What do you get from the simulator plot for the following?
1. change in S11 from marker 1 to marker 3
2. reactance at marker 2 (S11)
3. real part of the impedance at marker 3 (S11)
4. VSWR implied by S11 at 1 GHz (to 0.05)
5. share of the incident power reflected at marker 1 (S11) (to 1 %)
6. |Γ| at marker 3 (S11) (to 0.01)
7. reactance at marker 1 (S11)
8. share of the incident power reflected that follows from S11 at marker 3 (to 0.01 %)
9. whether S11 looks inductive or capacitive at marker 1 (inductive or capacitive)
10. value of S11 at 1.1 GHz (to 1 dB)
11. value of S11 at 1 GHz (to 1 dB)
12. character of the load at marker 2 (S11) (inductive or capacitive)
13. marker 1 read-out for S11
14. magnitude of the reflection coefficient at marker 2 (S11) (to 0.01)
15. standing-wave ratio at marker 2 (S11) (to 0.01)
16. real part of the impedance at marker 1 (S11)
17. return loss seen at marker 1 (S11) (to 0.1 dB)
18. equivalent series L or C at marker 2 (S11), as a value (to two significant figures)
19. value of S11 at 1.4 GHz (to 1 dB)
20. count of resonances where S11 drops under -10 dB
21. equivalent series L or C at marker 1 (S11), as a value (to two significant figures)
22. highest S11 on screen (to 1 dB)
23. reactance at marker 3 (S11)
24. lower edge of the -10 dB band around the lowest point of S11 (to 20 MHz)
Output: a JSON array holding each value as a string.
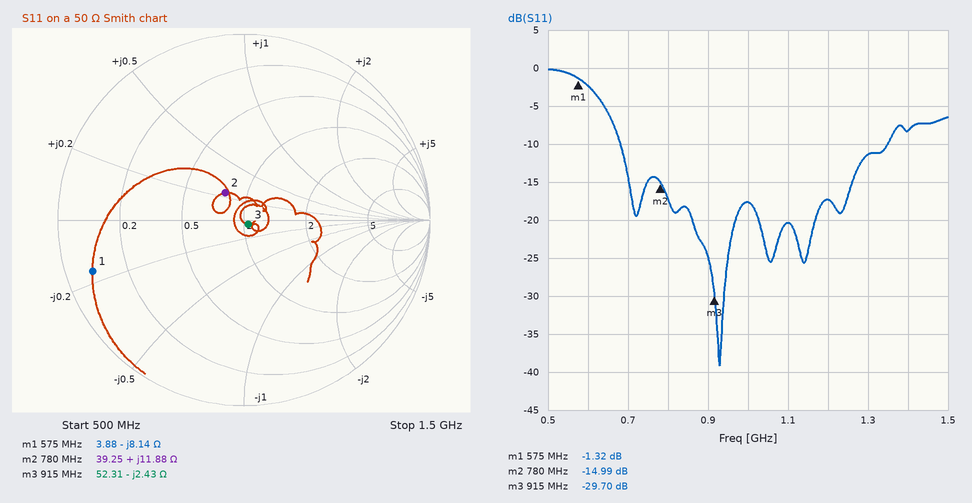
["-28.38 dB", "+11.88 Ω", "52.31 Ω", "1.30", "74 %", "0.03", "-8.14 Ω", "0.11 %", "capacitive", "-20 dB", "-18 dB", "inductive", "-1.32 dB", "0.18", "1.43", "3.88 Ω", "1.3 dB", "2.4 nH", "-8 dB", "4", "34 pF", "0 dB", "-2.43 Ω", "680 MHz"]
